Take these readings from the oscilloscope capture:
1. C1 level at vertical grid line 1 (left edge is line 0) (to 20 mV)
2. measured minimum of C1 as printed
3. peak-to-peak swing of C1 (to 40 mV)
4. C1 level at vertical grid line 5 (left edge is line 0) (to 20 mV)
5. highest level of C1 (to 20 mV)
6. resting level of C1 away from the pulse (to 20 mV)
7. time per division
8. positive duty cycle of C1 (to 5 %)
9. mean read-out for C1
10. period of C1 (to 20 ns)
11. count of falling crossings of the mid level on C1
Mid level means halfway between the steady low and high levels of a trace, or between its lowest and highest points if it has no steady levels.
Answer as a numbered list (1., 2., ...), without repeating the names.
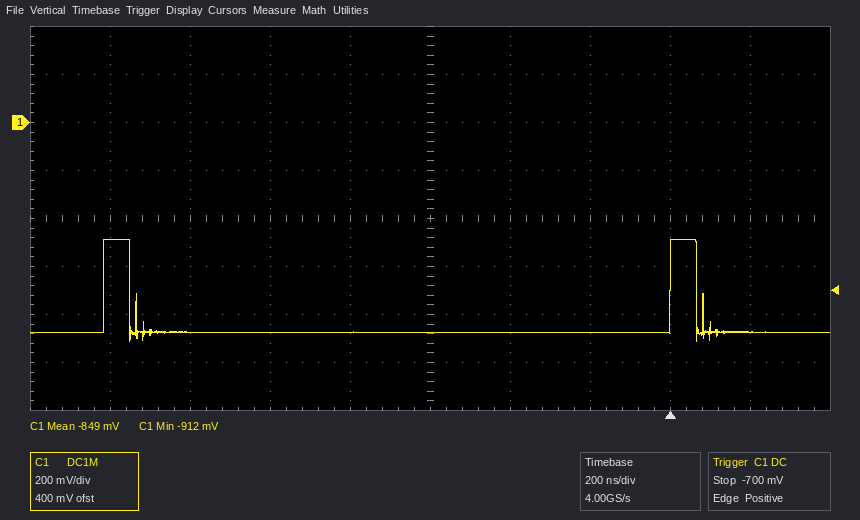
1. -480 mV
2. -912 mV
3. 440 mV
4. -880 mV
5. -480 mV
6. -880 mV
7. 200 ns
8. 5 %
9. -849 mV
10. 1.42 µs
11. 2
